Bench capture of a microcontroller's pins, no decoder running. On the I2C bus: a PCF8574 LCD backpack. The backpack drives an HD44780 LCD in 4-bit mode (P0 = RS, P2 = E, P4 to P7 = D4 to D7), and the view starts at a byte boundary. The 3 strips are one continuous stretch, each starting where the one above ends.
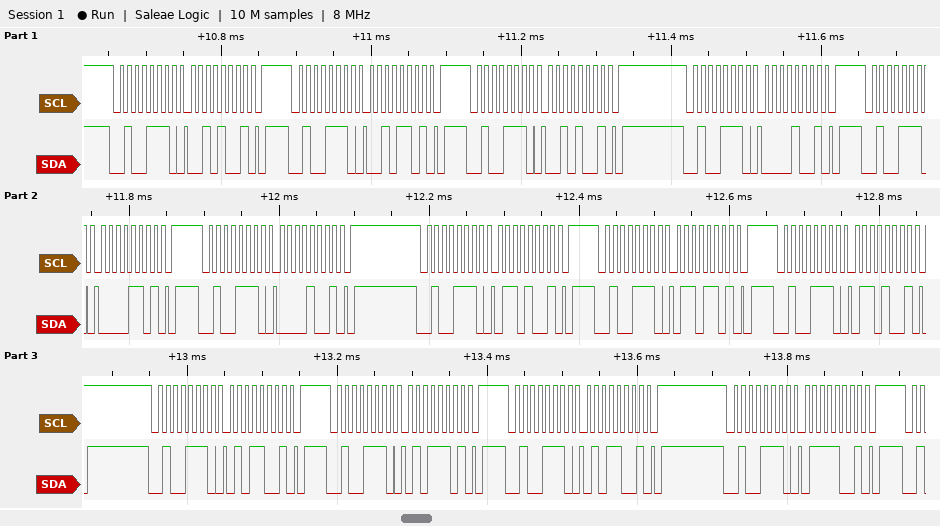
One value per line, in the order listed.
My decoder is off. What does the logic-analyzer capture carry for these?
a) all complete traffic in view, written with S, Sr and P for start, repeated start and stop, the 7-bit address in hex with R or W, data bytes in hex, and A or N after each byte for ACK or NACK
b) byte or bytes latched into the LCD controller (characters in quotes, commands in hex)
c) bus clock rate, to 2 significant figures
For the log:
S 27W A 29 A P S 27W A 2D A P S 27W A 29 A P S 27W A 09 A P S 27W A 0D A P S 27W A 09 A P S 27W A 69 A P S 27W A 6D A P S 27W A 69 A P S 27W A 59 A P S 27W A 5D A P S 27W A 59 A P S 27W A 79 A P
' ' 'e'
100 kHz
